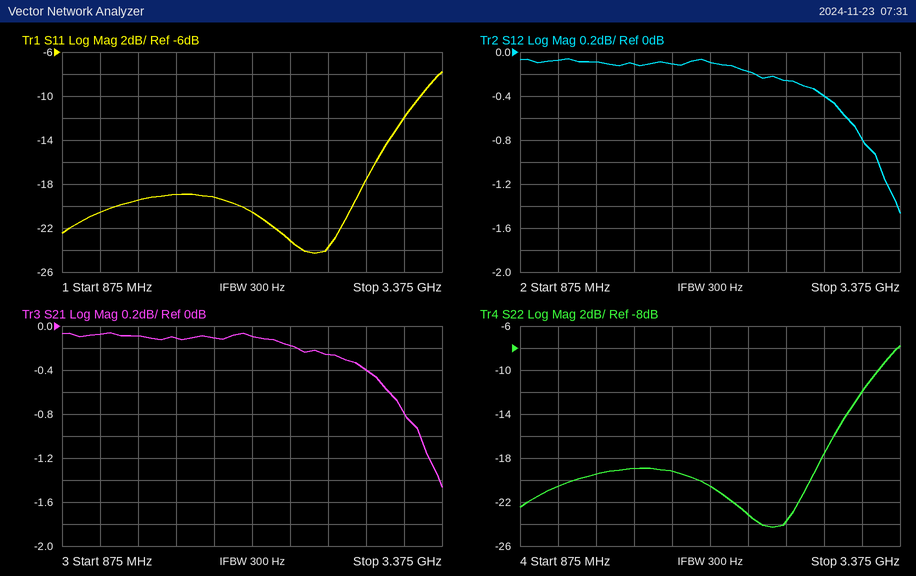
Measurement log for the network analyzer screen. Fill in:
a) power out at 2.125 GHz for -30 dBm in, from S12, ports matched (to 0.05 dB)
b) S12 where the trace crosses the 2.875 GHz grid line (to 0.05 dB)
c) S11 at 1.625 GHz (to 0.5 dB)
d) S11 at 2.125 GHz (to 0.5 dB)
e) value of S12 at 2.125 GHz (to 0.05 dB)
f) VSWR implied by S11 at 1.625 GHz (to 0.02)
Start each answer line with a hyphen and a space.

- -30.10 dBm
- -0.40 dB
- -19.0 dB
- -20.5 dB
- -0.10 dB
- 1.26
